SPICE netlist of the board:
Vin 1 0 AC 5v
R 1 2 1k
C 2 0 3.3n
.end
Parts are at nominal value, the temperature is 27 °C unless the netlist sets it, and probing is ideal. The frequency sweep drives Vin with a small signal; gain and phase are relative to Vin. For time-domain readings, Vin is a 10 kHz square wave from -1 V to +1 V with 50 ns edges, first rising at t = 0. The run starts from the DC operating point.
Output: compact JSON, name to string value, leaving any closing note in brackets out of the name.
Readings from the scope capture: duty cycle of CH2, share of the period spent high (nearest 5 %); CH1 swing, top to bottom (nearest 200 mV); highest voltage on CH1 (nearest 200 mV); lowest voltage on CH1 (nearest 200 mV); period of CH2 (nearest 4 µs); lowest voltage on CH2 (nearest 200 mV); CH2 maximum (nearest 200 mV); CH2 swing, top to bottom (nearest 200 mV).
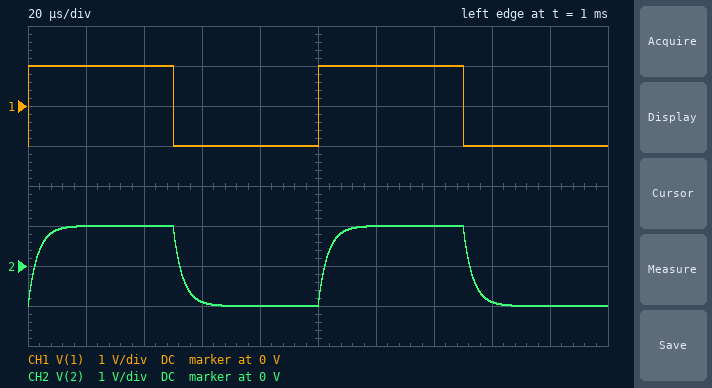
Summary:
{"duty cycle of CH2, share of the period spent high": "50 %", "CH1 swing, top to bottom": "2.0 V", "highest voltage on CH1": "1.0 V", "lowest voltage on CH1": "-1.0 V", "period of CH2": "100 µs", "lowest voltage on CH2": "-1.0 V", "CH2 maximum": "1.0 V", "CH2 swing, top to bottom": "2.0 V"}
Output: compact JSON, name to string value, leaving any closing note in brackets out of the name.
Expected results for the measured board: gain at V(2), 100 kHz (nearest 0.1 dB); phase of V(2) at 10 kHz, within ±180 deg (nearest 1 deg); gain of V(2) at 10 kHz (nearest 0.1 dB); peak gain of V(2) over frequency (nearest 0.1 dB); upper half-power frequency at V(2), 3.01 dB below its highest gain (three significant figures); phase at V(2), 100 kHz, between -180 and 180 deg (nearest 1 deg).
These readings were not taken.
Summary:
{"gain at V(2), 100 kHz": "-7.2 dB", "phase of V(2) at 10 kHz, within ±180 deg": "-12 deg", "gain of V(2) at 10 kHz": "-0.2 dB", "peak gain of V(2) over frequency": "0 dB", "upper half-power frequency at V(2), 3.01 dB below its highest gain": "48.2 kHz", "phase at V(2), 100 kHz, between -180 and 180 deg": "-64 deg"}
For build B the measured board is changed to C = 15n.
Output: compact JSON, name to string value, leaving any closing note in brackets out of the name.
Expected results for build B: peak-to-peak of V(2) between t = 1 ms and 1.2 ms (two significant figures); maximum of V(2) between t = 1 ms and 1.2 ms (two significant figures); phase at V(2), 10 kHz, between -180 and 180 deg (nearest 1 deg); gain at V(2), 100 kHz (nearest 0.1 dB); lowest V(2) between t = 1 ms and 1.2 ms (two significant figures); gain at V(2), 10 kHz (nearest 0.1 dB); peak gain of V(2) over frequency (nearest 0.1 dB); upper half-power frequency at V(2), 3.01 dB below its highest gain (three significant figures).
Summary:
{"peak-to-peak of V(2) between t = 1 ms and 1.2 ms": "1.9 V", "maximum of V(2) between t = 1 ms and 1.2 ms": "930 mV", "phase at V(2), 10 kHz, between -180 and 180 deg": "-43 deg", "gain at V(2), 100 kHz": "-19.5 dB", "lowest V(2) between t = 1 ms and 1.2 ms": "-930 mV", "gain at V(2), 10 kHz": "-2.8 dB", "peak gain of V(2) over frequency": "0 dB", "upper half-power frequency at V(2), 3.01 dB below its highest gain": "10.6 kHz"}
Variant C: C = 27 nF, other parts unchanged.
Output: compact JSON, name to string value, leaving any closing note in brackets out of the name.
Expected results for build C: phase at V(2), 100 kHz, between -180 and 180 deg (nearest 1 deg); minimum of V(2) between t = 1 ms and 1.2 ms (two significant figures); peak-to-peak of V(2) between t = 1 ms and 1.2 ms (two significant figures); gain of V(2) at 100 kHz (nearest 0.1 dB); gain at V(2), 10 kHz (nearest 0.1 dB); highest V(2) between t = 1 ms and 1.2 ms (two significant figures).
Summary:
{"phase at V(2), 100 kHz, between -180 and 180 deg": "-87 deg", "minimum of V(2) between t = 1 ms and 1.2 ms": "-730 mV", "peak-to-peak of V(2) between t = 1 ms and 1.2 ms": "1.5 V", "gain of V(2) at 100 kHz": "-24.6 dB", "gain at V(2), 10 kHz": "-5.9 dB", "highest V(2) between t = 1 ms and 1.2 ms": "730 mV"}
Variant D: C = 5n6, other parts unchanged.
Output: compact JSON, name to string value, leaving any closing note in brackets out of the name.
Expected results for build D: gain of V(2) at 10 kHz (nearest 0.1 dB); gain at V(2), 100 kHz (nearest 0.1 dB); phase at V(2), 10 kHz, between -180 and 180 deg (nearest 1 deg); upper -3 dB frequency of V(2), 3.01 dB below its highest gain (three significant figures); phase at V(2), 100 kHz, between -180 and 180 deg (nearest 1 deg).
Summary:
{"gain of V(2) at 10 kHz": "-0.5 dB", "gain at V(2), 100 kHz": "-11.3 dB", "phase at V(2), 10 kHz, between -180 and 180 deg": "-19 deg", "upper -3 dB frequency of V(2), 3.01 dB below its highest gain": "28.4 kHz", "phase at V(2), 100 kHz, between -180 and 180 deg": "-74 deg"}
